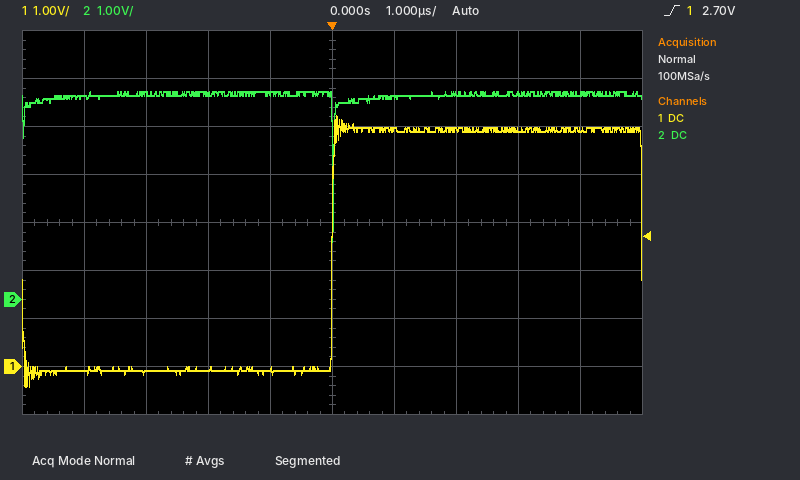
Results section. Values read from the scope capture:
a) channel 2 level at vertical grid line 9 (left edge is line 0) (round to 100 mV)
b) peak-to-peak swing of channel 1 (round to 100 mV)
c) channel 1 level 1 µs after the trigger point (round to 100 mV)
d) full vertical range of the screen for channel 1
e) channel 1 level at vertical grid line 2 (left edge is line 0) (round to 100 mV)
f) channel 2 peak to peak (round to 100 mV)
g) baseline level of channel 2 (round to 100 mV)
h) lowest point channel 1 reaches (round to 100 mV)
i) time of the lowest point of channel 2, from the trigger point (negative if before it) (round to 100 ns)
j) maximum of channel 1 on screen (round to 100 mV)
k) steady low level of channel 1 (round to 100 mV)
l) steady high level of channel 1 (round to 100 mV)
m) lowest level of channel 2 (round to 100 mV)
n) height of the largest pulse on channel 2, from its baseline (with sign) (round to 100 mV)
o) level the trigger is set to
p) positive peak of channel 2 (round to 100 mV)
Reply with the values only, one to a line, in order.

4.3 V
5.6 V
4.9 V
8 V
-100 mV
3.1 V
4.3 V
-400 mV
0.0 µs
5.2 V
-100 mV
4.9 V
1.2 V
-3.1 V
2.70 V
4.3 V
